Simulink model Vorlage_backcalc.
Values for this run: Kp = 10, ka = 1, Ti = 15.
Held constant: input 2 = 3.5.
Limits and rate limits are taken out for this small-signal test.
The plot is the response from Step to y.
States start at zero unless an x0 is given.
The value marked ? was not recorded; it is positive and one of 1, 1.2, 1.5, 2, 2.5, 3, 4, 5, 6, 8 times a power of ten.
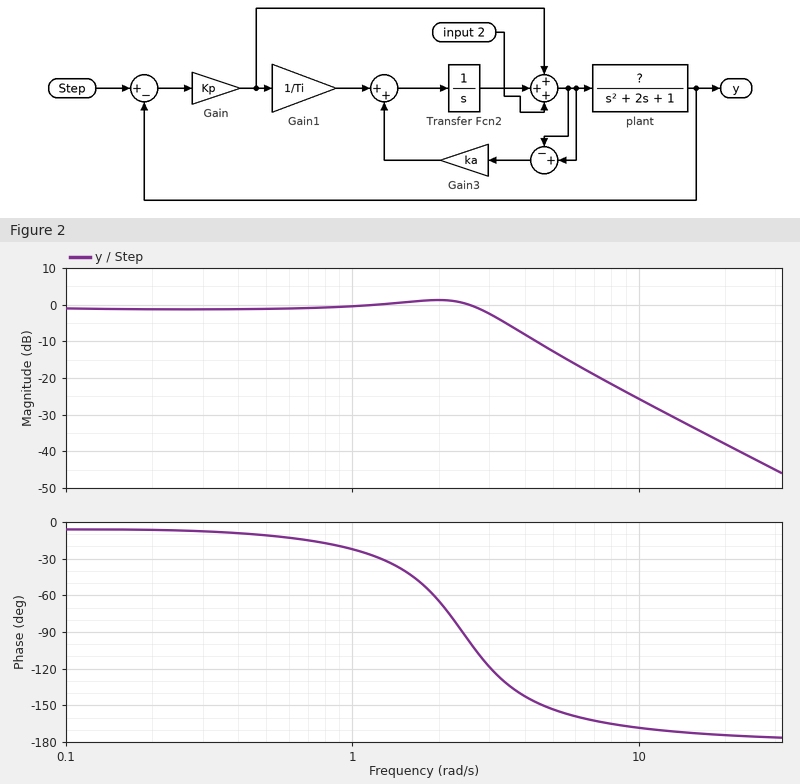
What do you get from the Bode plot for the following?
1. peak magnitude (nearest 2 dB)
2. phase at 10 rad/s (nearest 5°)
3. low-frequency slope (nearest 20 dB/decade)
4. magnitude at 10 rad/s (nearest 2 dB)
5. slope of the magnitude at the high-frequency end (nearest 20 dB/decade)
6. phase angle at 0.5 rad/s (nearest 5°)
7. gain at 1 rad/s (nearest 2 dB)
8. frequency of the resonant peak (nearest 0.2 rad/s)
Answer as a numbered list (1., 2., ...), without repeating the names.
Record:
1. 2 dB
2. -170°
3. 0 dB/decade
4. -26 dB
5. -40 dB/decade
6. -10°
7. 0 dB
8. 2.0 rad/s
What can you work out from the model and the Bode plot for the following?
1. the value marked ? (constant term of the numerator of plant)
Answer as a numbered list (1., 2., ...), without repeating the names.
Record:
1. 0.5
